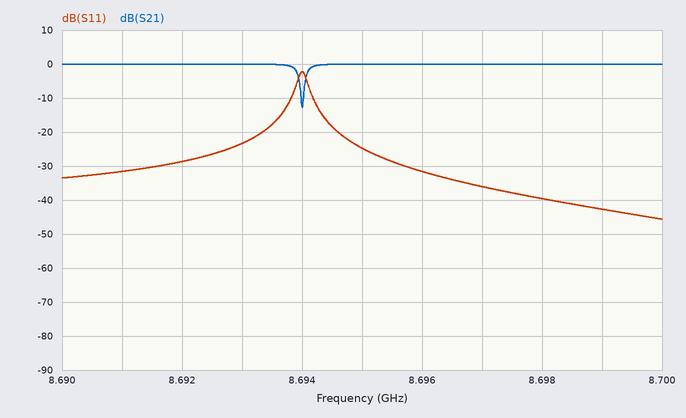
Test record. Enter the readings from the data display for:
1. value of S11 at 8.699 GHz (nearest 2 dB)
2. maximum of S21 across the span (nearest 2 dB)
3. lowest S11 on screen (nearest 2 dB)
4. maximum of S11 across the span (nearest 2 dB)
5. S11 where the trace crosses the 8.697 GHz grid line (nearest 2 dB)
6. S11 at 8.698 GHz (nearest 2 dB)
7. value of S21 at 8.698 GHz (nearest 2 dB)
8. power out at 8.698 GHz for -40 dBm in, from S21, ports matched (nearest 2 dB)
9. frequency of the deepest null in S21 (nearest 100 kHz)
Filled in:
-42 dB
0 dB
-46 dB
-2 dB
-36 dB
-40 dB
0 dB
-40 dBm
8.6940 GHz
